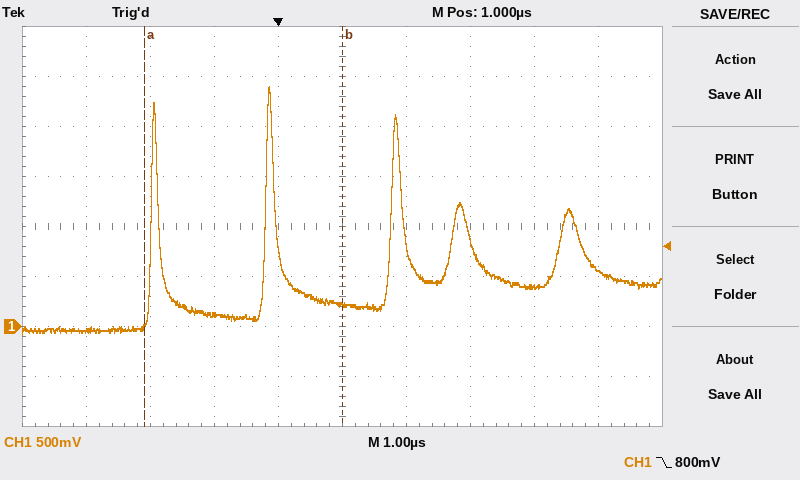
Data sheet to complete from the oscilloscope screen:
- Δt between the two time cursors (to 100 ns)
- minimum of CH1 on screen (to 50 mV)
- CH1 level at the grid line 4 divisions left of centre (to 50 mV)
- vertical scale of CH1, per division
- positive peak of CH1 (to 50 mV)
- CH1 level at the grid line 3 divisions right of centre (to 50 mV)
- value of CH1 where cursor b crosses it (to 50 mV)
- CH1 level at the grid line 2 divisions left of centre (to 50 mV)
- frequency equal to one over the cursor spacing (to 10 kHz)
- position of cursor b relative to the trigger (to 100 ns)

3.1 µs
-100 mV
-50 mV
500 mV
2.40 V
400 mV
200 mV
100 mV
320 kHz
+1.0 µs
